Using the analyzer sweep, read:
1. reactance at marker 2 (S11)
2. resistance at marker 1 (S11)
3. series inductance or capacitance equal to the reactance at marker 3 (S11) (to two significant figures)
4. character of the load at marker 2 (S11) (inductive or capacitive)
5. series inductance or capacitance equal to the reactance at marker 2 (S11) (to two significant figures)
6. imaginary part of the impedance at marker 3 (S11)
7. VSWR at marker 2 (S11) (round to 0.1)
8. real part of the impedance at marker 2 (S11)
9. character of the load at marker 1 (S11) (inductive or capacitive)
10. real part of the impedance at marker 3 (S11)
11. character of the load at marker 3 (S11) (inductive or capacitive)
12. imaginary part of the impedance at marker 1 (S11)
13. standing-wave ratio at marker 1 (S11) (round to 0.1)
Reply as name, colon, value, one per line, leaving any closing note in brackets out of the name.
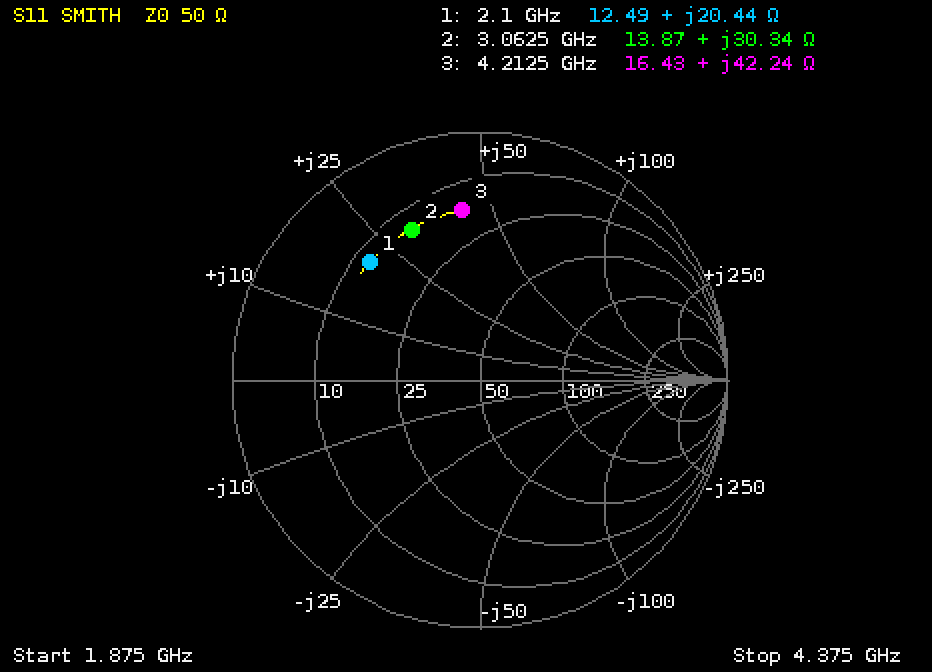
reactance at marker 2: +30.34 Ω
resistance at marker 1: 12.49 Ω
series inductance or capacitance equal to the reactance at marker 3 (S11): 1.6 nH
character of the load at marker 2 (S11): inductive
series inductance or capacitance equal to the reactance at marker 2 (S11): 1.6 nH
imaginary part of the impedance at marker 3: +42.24 Ω
VSWR at marker 2 (S11): 5.0
real part of the impedance at marker 2: 13.87 Ω
character of the load at marker 1 (S11): inductive
real part of the impedance at marker 3: 16.43 Ω
character of the load at marker 3 (S11): inductive
imaginary part of the impedance at marker 1: +20.44 Ω
standing-wave ratio at marker 1 (S11): 4.7
